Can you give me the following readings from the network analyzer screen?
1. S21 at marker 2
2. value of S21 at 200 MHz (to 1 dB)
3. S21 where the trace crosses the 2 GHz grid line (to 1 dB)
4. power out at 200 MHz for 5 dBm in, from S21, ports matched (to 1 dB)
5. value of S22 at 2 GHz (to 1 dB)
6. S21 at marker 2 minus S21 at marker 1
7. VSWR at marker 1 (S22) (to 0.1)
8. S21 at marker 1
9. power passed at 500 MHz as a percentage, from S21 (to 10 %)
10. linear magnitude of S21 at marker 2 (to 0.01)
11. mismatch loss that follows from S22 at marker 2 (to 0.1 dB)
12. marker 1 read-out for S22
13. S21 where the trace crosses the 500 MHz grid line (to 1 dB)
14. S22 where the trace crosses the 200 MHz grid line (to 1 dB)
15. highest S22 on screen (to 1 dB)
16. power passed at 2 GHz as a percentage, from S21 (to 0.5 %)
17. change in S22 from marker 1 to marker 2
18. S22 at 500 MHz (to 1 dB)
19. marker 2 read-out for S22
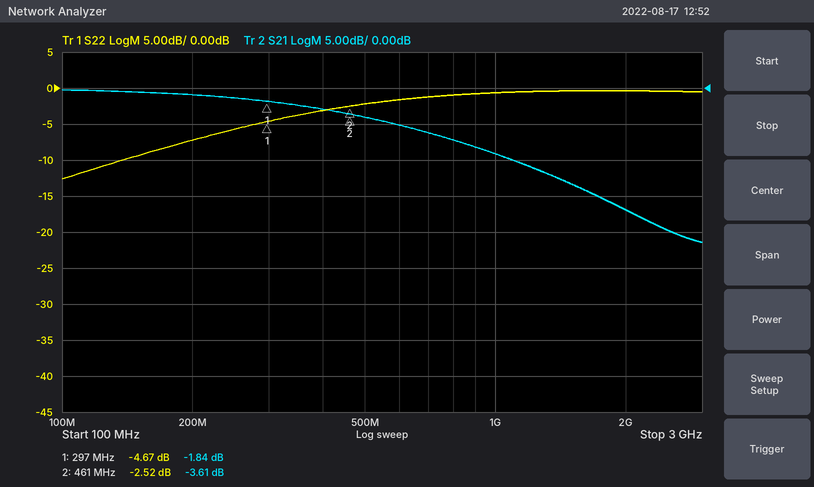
-3.61 dB
-1 dB
-17 dB
4 dBm
0 dB
-1.77 dB
3.8
-1.84 dB
40 %
0.66
3.6 dB
-4.67 dB
-4 dB
-7 dB
0 dB
2.0 %
2.15 dB
-2 dB
-2.52 dB
